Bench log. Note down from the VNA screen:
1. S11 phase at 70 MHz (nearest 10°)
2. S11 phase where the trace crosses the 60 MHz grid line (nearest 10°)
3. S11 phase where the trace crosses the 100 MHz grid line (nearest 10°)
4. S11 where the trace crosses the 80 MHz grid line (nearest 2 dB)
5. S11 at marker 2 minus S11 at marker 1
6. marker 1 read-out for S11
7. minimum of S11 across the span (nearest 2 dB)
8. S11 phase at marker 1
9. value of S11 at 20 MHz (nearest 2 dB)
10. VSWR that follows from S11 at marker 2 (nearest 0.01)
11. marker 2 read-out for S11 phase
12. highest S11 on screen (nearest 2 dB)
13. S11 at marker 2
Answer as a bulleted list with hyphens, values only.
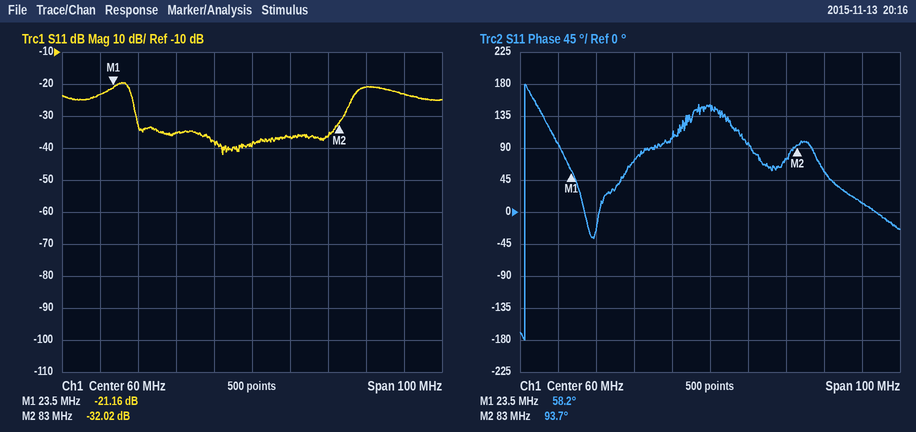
- 100°
- 150°
- 10°
- -36 dB
- -10.86 dB
- -21.16 dB
- -42 dB
- 58.2°
- -24 dB
- 1.05
- 93.7°
- -20 dB
- -32.02 dB
